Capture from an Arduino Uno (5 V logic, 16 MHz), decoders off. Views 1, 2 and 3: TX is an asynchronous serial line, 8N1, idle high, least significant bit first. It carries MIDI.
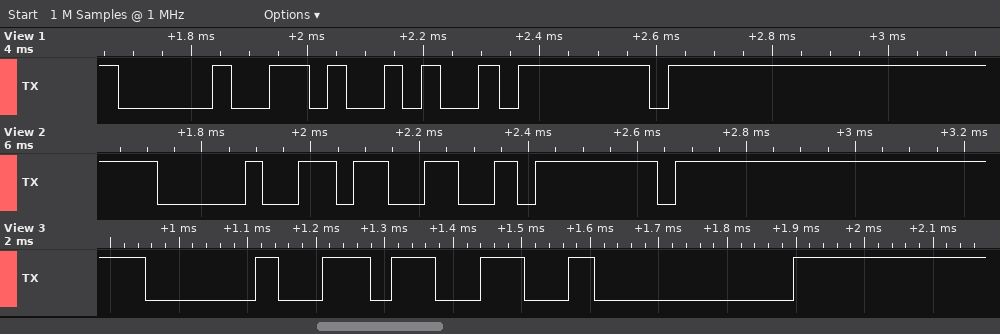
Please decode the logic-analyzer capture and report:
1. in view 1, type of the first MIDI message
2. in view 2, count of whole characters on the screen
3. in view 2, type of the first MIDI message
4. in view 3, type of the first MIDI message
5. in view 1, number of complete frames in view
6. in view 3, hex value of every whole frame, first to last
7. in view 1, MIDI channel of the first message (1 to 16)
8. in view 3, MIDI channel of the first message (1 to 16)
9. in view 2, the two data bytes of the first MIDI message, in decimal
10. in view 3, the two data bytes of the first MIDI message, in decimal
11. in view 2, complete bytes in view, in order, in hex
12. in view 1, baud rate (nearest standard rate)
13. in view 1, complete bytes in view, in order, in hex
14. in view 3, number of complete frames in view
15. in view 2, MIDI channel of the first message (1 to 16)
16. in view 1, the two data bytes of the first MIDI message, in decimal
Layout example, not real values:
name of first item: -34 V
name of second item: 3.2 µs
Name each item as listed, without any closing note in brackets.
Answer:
in view 1, type of the first MIDI message: Note On
in view 2, count of whole characters on the screen: 3
in view 2, type of the first MIDI message: Note On
in view 3, type of the first MIDI message: Note On
in view 1, number of complete frames in view: 3
in view 3, hex value of every whole frame, first to last: 90 33 00
in view 1, MIDI channel of the first message: 1
in view 3, MIDI channel of the first message: 1
in view 2, the two data bytes of the first MIDI message, in decimal: 51, 127
in view 3, the two data bytes of the first MIDI message, in decimal: 51, 0
in view 2, complete bytes in view, in order, in hex: 90 33 7F
in view 1, baud rate: 31250 baud
in view 1, complete bytes in view, in order, in hex: 90 29 7F
in view 3, number of complete frames in view: 3
in view 2, MIDI channel of the first message: 1
in view 1, the two data bytes of the first MIDI message, in decimal: 41, 127
